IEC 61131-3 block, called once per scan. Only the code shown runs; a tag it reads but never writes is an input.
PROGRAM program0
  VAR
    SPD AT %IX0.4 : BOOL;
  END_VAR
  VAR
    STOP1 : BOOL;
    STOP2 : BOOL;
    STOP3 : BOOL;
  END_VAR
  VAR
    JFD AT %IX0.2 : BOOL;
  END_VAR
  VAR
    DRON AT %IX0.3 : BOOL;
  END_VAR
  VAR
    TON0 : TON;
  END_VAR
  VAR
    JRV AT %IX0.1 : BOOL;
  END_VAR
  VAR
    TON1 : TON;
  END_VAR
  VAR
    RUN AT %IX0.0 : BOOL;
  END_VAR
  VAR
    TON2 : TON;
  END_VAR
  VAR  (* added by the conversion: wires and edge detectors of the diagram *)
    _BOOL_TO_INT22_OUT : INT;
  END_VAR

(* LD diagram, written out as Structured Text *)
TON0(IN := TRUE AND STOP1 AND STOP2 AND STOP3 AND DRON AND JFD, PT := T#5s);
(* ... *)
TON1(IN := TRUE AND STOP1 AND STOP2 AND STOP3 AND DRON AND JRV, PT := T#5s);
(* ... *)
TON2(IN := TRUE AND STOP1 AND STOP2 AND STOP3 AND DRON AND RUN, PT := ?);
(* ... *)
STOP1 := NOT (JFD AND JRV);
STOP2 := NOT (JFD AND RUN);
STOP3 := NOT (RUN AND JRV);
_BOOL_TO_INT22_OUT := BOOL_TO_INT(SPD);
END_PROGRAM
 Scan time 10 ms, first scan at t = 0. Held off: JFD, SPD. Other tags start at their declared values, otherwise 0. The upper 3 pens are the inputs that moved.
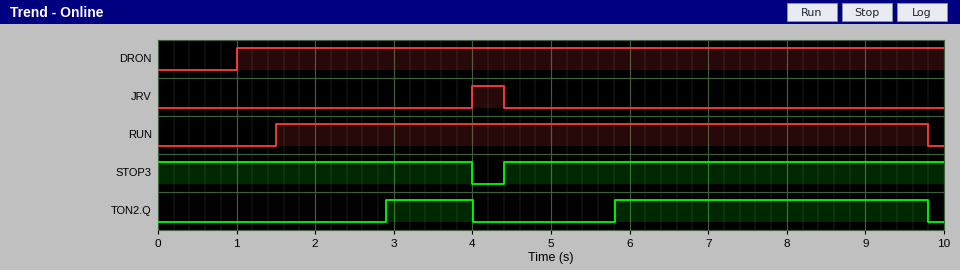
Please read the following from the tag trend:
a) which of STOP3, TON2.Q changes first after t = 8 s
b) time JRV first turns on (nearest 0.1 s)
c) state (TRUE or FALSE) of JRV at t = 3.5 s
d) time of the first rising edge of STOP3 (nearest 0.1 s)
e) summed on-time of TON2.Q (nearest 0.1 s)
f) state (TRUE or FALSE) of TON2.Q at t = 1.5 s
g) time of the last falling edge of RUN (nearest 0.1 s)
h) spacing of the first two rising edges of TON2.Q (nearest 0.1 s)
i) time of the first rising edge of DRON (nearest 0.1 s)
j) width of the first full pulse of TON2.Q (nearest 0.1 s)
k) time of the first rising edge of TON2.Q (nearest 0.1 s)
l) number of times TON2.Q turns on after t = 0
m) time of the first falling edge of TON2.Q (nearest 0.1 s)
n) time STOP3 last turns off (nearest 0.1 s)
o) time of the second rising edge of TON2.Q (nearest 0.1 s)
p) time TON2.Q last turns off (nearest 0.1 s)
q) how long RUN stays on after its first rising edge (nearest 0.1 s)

TON2.Q
4.0 s
FALSE
4.4 s
5.1 s
FALSE
9.8 s
2.9 s
1.0 s
1.1 s
2.9 s
2
4.0 s
4.0 s
5.8 s
9.8 s
8.3 s
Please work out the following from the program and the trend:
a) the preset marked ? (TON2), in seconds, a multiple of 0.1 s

1.4 s
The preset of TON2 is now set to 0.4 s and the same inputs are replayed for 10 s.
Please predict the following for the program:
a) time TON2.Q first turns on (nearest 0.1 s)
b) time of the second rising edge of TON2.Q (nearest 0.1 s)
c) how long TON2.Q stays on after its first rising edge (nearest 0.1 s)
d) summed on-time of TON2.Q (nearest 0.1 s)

1.9 s
4.8 s
2.1 s
7.1 s
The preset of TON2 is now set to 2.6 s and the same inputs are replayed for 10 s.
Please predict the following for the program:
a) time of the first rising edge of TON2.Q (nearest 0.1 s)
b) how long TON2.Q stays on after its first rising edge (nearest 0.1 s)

7.0 s
2.8 s
